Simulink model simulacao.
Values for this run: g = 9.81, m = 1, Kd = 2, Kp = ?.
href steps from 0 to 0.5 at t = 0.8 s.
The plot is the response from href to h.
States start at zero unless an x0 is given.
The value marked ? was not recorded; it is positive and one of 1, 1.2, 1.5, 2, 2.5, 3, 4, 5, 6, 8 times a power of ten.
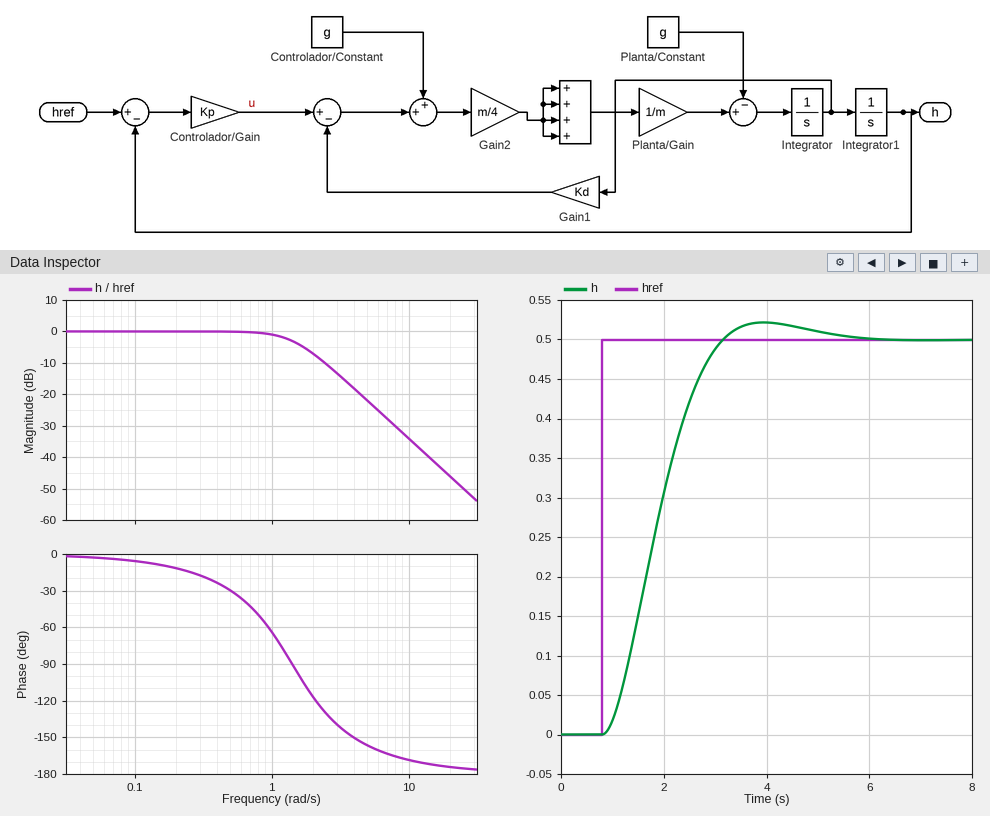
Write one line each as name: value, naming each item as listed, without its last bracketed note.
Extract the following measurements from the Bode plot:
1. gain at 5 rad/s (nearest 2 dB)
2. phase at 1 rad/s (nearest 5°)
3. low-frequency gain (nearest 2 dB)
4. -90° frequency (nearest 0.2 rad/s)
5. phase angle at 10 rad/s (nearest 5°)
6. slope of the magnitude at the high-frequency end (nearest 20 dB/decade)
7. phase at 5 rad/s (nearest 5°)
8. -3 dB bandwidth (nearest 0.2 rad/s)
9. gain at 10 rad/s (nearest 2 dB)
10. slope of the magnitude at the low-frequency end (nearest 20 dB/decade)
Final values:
gain at 5 rad/s: -22 dB
phase at 1 rad/s: -65°
low-frequency gain: 0 dB
-90° frequency: 1.4 rad/s
phase angle at 10 rad/s: -170°
slope of the magnitude at the high-frequency end: -40 dB/decade
phase at 5 rad/s: -155°
-3 dB bandwidth: 1.4 rad/s
gain at 10 rad/s: -34 dB
slope of the magnitude at the low-frequency end: 0 dB/decade
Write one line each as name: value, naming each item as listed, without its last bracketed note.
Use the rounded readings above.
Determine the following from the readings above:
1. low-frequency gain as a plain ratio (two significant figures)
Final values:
low-frequency gain as a plain ratio: 1.0
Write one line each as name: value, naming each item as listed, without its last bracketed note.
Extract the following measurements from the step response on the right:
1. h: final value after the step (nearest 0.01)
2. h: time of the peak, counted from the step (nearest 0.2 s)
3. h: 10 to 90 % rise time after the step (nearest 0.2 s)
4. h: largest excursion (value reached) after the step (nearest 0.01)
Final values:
h: final value after the step: 0.50
h: time of the peak, counted from the step: 3.2 s
h: 10 to 90 % rise time after the step: 1.6 s
h: largest excursion (value reached) after the step: 0.52
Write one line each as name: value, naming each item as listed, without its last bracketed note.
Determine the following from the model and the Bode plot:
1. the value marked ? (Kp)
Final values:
the value marked ?: 2
